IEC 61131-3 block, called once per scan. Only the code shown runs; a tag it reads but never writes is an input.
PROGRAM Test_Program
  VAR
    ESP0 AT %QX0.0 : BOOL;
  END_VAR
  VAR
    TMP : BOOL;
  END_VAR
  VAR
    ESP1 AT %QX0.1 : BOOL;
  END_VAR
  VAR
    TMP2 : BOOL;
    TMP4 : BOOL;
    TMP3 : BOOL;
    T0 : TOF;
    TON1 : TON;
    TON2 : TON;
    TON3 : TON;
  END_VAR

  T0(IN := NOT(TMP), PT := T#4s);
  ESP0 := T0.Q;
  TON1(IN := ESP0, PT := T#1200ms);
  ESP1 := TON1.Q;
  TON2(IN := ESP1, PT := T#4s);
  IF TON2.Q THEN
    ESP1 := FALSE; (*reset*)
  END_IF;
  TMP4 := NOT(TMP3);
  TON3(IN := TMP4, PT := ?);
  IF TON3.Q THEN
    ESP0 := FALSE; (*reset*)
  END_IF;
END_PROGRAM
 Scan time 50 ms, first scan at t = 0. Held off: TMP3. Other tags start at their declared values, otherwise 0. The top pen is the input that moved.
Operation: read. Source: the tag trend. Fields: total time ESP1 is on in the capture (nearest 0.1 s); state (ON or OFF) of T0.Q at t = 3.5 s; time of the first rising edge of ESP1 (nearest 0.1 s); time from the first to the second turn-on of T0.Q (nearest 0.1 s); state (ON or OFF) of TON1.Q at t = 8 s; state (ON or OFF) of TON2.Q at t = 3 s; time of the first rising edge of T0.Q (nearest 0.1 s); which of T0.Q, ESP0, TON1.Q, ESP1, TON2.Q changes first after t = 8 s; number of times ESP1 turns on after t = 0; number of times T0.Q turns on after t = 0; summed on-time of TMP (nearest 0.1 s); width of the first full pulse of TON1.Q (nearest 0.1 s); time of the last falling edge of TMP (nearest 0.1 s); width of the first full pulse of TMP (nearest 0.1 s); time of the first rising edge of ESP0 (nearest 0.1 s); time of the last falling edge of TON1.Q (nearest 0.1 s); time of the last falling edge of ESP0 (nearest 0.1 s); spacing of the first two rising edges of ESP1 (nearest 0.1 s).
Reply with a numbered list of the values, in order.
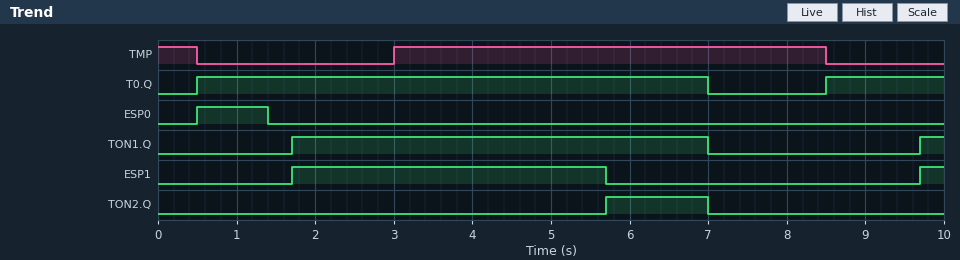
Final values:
1. 4.3 s
2. ON
3. 1.7 s
4. 8.0 s
5. OFF
6. OFF
7. 0.5 s
8. T0.Q
9. 2
10. 2
11. 6.0 s
12. 5.3 s
13. 8.5 s
14. 5.5 s
15. 0.5 s
16. 7.0 s
17. 1.4 s
18. 8.0 s
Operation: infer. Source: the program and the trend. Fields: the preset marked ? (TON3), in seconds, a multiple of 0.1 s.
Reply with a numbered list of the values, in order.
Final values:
1. 1.4 s
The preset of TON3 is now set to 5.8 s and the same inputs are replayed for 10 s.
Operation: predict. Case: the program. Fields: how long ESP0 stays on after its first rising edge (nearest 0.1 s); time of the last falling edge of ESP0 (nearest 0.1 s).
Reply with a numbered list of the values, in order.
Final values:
1. 5.3 s
2. 5.8 s
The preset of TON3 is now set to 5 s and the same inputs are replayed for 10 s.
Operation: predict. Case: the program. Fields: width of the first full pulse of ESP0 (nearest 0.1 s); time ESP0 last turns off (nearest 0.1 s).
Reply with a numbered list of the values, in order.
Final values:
1. 4.5 s
2. 5.0 s
